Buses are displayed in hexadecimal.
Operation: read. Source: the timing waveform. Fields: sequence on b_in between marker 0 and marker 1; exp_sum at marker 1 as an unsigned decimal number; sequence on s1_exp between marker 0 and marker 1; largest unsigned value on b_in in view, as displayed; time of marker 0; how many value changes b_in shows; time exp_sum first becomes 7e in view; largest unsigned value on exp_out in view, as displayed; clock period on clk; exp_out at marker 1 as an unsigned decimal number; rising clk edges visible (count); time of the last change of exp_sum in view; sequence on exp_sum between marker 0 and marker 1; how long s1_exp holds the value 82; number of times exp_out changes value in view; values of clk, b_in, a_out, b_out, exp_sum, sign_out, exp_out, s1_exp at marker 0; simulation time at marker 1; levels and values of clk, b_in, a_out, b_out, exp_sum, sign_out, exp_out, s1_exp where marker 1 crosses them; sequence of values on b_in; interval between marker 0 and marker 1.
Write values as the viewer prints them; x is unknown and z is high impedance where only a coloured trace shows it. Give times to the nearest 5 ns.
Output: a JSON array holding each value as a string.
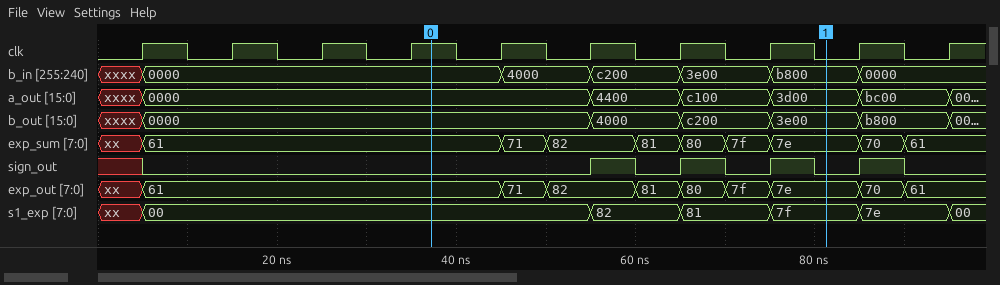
["0000, 4000, c200, 3e00, b800", "126", "00, 82, 81, 7f", "c200", "35 ns", "6", "75 ns", "82", "10 ns", "126", "10", "90 ns", "61, 71, 82, 81, 80, 7f, 7e", "10 ns", "9", "clk=1, b_in=0000, a_out=0000, b_out=0000, exp_sum=61, sign_out=0, exp_out=61, s1_exp=00", "80 ns", "clk=0, b_in=b800, a_out=3d00, b_out=3e00, exp_sum=7e, sign_out=0, exp_out=7e, s1_exp=7f", "xxxx, 0000, 4000, c200, 3e00, b800, 0000", "45 ns"]
